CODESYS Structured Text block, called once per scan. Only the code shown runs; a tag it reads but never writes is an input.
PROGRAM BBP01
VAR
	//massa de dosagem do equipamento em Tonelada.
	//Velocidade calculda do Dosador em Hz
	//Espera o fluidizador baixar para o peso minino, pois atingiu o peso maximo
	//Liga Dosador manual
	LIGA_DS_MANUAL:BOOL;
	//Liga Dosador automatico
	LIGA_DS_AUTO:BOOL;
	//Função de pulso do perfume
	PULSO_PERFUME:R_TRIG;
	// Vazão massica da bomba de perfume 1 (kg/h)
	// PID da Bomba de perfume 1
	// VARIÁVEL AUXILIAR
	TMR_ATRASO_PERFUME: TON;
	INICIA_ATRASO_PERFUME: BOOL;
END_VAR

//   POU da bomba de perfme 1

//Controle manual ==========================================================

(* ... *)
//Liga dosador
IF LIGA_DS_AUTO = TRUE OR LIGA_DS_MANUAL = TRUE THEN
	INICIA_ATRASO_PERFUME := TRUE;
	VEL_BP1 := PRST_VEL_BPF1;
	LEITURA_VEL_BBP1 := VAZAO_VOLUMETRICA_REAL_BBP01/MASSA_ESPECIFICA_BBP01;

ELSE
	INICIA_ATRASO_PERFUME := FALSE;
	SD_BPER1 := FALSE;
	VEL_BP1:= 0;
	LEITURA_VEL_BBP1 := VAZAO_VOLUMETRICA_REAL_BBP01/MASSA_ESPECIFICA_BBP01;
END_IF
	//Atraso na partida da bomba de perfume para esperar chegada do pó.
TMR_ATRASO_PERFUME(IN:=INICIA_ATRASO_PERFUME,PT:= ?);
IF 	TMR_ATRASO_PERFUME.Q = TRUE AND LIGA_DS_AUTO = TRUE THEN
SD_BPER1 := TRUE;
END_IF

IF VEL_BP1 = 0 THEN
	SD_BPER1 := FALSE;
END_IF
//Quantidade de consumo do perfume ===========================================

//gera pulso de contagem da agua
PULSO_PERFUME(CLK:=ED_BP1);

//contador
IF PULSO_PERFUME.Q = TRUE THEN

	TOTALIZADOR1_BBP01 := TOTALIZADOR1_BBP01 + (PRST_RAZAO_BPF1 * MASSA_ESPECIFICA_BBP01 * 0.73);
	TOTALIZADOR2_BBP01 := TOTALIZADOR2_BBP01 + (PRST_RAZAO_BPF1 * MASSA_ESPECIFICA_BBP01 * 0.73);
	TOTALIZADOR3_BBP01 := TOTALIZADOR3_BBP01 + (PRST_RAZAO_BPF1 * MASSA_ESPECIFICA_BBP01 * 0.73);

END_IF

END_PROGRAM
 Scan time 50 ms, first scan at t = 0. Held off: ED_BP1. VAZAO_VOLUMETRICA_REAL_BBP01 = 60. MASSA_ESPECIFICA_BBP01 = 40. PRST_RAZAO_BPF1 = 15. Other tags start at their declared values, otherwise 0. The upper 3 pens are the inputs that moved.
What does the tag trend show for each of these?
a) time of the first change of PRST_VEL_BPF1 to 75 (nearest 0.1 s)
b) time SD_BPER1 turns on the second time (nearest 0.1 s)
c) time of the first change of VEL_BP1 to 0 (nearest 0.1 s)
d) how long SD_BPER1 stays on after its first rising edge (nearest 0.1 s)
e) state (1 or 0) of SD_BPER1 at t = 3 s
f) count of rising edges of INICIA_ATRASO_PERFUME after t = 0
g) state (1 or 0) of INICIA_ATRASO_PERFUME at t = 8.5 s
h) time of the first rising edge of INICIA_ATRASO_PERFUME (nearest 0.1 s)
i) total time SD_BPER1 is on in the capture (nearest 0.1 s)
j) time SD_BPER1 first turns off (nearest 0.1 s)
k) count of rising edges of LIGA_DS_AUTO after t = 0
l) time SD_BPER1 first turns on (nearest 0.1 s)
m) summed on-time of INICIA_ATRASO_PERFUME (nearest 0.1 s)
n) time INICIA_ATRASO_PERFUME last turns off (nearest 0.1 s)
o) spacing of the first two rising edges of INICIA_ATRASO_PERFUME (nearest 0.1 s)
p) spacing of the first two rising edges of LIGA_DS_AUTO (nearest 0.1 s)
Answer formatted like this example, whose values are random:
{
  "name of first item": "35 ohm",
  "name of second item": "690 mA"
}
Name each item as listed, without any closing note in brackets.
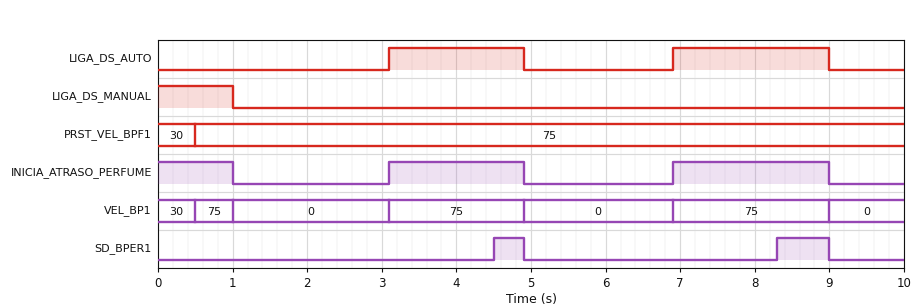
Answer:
{
  "time of the first change of PRST_VEL_BPF1 to 75": "0.5 s",
  "time SD_BPER1 turns on the second time": "8.3 s",
  "time of the first change of VEL_BP1 to 0": "1.0 s",
  "how long SD_BPER1 stays on after its first rising edge": "0.4 s",
  "state (1 or 0) of SD_BPER1 at t = 3 s": "0",
  "count of rising edges of INICIA_ATRASO_PERFUME after t = 0": "2",
  "state (1 or 0) of INICIA_ATRASO_PERFUME at t = 8.5 s": "1",
  "time of the first rising edge of INICIA_ATRASO_PERFUME": "3.1 s",
  "total time SD_BPER1 is on in the capture": "1.1 s",
  "time SD_BPER1 first turns off": "4.9 s",
  "count of rising edges of LIGA_DS_AUTO after t = 0": "2",
  "time SD_BPER1 first turns on": "4.5 s",
  "summed on-time of INICIA_ATRASO_PERFUME": "4.9 s",
  "time INICIA_ATRASO_PERFUME last turns off": "9.0 s",
  "spacing of the first two rising edges of INICIA_ATRASO_PERFUME": "3.8 s",
  "spacing of the first two rising edges of LIGA_DS_AUTO": "3.8 s"
}
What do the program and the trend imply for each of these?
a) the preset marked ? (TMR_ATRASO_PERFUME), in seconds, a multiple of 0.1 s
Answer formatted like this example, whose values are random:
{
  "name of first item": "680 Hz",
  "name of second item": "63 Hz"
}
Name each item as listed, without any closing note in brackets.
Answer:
{
  "the preset marked ? (TMR_ATRASO_PERFUME), in seconds, a multiple of 0.1 s": "1.4 s"
}
